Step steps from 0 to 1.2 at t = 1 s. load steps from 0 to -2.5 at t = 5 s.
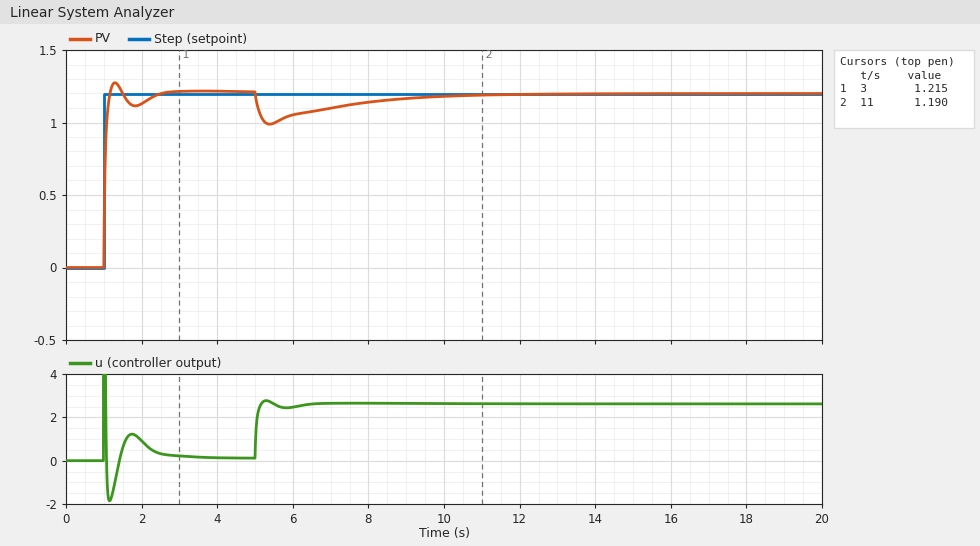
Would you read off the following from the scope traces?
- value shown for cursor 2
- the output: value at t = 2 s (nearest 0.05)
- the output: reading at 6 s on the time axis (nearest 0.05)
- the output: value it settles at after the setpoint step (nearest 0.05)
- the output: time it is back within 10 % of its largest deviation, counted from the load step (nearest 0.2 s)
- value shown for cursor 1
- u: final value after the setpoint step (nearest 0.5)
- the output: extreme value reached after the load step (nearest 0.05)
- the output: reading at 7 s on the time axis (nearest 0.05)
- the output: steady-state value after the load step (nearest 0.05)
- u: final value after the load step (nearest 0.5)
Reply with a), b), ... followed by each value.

a) 1.190
b) 1.15
c) 1.05
d) 1.20
e) 4.8 s
f) 1.215
g) 0.0
h) 1.00
i) 1.10
j) 1.20
k) 2.5
